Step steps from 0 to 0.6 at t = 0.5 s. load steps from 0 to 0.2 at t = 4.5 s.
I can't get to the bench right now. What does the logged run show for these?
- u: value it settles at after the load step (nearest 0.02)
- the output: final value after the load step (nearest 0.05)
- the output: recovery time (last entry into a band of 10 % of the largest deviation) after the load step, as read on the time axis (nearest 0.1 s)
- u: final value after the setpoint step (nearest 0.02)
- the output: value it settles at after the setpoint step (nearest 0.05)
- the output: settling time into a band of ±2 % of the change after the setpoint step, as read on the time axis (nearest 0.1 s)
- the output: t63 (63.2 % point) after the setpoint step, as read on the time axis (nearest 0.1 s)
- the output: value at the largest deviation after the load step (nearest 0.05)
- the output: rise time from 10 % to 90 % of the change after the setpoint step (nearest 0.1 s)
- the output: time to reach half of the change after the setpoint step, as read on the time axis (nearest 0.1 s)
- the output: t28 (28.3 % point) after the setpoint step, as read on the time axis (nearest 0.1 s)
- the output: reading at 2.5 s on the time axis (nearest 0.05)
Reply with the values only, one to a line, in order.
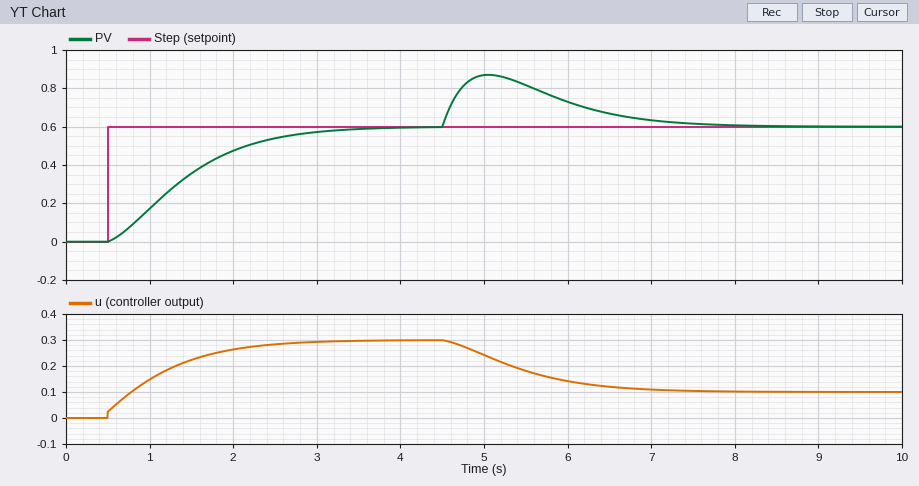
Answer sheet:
0.10
0.60
7.1 s
0.30
0.60
3.5 s
1.6 s
0.85
1.8 s
1.3 s
1.0 s
0.55
